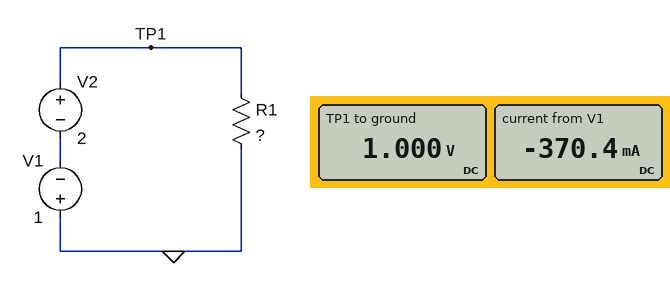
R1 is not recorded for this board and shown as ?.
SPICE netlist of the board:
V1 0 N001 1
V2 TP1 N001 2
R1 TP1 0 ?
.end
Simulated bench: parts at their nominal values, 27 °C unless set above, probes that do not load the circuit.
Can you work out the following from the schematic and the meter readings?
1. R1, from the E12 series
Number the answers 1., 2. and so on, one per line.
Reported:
1. 2.7 Ω
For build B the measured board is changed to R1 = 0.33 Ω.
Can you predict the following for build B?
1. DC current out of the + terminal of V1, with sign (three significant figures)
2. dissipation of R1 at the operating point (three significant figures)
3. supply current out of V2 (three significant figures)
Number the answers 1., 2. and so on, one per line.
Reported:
1. -3.03 A
2. 3.03 W
3. 3.03 A
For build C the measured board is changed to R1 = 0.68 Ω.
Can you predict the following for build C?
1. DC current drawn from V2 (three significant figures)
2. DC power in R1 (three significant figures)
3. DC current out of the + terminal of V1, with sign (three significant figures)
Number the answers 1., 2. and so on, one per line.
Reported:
1. 1.47 A
2. 1.47 W
3. -1.47 A
